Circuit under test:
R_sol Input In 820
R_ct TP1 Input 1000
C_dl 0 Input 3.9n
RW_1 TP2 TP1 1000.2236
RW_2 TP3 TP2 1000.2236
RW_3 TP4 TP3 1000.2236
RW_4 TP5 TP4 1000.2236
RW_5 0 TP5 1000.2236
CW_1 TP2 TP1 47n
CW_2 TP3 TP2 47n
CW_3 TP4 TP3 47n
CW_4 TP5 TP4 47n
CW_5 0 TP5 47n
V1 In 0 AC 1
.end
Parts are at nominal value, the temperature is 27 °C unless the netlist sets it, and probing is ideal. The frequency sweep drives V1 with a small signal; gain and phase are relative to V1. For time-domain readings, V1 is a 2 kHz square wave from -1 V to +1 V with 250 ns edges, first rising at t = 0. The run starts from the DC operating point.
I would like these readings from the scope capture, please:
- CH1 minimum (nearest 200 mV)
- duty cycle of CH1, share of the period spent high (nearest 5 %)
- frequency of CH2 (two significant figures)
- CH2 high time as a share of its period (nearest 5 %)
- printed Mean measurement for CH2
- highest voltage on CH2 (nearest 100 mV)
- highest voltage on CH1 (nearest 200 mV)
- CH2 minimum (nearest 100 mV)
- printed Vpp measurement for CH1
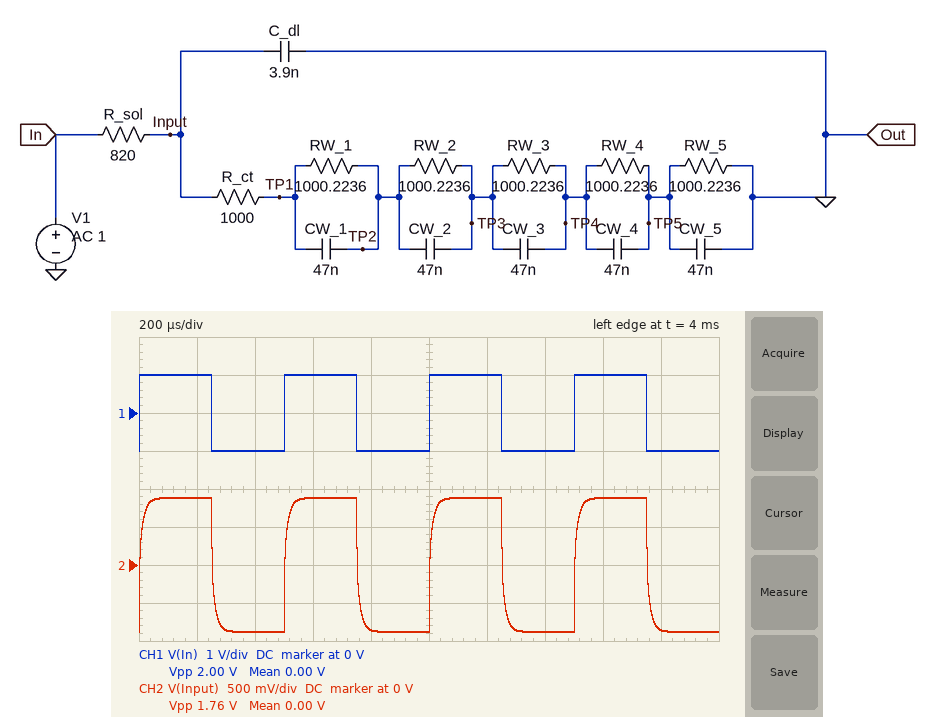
-1.0 V
50 %
2.0 kHz
50 %
0.00 V
900 mV
1.0 V
-900 mV
2.00 V
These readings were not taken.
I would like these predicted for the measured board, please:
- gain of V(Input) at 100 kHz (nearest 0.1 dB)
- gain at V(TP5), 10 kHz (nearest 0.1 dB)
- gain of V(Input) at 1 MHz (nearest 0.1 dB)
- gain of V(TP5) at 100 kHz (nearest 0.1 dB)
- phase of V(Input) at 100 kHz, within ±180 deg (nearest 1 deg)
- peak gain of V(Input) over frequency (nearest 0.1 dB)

-8.9 dB
-19.1 dB
-26.1 dB
-38.5 dB
-50 deg
-1.1 dB
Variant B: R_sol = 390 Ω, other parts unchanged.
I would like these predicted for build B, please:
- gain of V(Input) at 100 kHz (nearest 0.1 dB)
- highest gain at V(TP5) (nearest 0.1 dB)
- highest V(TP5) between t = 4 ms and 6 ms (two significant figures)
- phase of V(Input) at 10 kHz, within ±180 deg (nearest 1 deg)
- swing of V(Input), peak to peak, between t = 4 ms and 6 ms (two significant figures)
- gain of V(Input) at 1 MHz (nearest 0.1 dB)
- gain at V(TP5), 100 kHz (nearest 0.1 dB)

-4.7 dB
-16.1 dB
160 mV
-11 deg
1.9 V
-19.7 dB
-34.3 dB
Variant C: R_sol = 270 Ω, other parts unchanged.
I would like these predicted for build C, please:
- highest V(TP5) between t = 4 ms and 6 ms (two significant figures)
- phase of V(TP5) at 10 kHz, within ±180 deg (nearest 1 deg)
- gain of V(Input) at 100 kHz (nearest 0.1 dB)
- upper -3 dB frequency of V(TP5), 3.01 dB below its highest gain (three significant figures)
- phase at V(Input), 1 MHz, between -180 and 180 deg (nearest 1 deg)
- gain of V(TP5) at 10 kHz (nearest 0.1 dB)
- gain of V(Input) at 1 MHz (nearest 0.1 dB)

160 mV
-34 deg
-3.2 dB
16.3 kHz
-79 deg
-17.3 dB
-16.6 dB
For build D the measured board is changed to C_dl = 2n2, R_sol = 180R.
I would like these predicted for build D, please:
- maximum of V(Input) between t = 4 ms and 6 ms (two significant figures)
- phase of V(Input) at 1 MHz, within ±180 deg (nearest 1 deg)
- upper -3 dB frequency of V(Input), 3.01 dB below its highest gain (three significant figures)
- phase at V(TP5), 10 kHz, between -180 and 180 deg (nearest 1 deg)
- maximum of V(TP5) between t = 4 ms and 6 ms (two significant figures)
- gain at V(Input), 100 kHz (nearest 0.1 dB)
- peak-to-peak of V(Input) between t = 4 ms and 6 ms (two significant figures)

970 mV
-65 deg
340 kHz
-31 deg
160 mV
-1.6 dB
1.9 V
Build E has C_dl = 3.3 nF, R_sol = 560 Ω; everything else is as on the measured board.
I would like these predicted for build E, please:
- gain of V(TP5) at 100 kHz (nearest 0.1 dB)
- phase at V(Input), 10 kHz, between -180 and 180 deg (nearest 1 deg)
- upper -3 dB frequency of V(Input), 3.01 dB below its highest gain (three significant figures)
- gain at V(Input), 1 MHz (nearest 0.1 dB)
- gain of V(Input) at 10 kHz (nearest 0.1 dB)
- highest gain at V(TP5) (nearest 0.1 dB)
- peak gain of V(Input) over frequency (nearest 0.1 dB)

-35.5 dB
-14 deg
32.7 kHz
-21.4 dB
-1.7 dB
-16.3 dB
-0.8 dB
